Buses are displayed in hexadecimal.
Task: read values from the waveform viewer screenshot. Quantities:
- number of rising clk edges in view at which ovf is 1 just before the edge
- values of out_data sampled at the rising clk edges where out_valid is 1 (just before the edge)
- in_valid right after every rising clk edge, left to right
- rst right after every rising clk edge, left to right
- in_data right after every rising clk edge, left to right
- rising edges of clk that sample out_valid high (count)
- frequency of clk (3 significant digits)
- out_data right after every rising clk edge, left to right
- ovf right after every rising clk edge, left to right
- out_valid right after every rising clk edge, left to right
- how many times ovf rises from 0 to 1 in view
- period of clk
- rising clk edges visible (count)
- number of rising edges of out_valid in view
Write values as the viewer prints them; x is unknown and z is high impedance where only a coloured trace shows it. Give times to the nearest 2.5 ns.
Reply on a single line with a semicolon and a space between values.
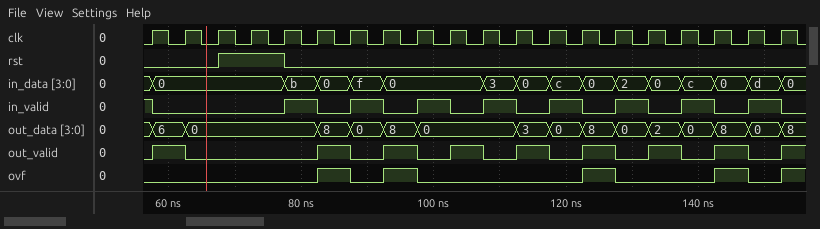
4; 6, 8, 8, 0, 3, 8, 2, 8; 0 0 0 0 1 0 1 0 1 0 1 0 1 0 1 0 1 0 1 0; 0 0 1 1 0 0 0 0 0 0 0 0 0 0 0 0 0 0 0 0; 0, 0, 0, 0, b, 0, f, 0, 0, 0, 3, 0, c, 0, 2, 0, c, 0, d, 0; 8; 200 MHz; 6, 0, 0, 0, 0, 8, 0, 8, 0, 0, 0, 3, 0, 8, 0, 2, 0, 8, 0, 8; 0 0 0 0 0 1 0 1 0 0 0 0 0 1 0 0 0 1 0 1; 1 0 0 0 0 1 0 1 0 1 0 1 0 1 0 1 0 1 0 1; 5; 5 ns; 20; 9
